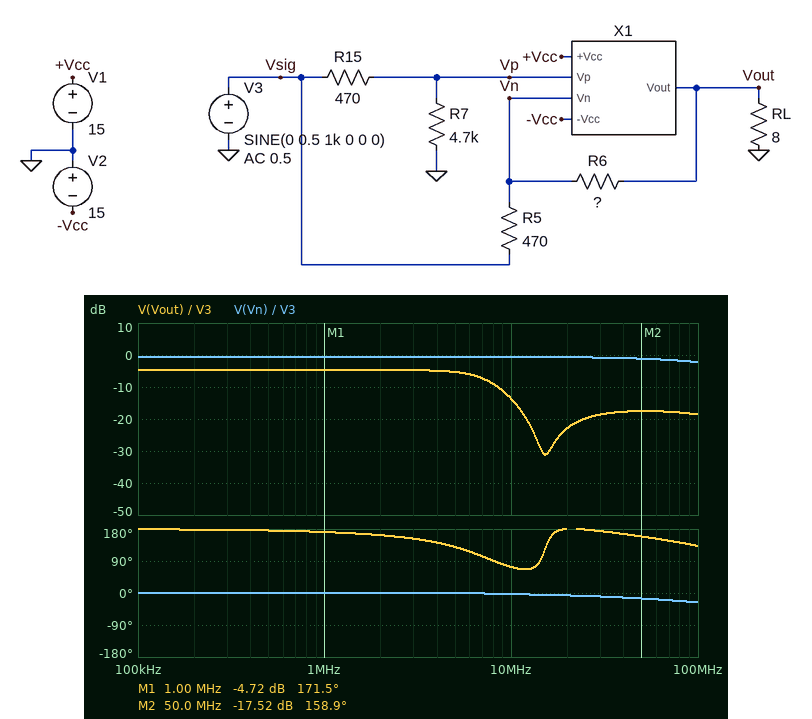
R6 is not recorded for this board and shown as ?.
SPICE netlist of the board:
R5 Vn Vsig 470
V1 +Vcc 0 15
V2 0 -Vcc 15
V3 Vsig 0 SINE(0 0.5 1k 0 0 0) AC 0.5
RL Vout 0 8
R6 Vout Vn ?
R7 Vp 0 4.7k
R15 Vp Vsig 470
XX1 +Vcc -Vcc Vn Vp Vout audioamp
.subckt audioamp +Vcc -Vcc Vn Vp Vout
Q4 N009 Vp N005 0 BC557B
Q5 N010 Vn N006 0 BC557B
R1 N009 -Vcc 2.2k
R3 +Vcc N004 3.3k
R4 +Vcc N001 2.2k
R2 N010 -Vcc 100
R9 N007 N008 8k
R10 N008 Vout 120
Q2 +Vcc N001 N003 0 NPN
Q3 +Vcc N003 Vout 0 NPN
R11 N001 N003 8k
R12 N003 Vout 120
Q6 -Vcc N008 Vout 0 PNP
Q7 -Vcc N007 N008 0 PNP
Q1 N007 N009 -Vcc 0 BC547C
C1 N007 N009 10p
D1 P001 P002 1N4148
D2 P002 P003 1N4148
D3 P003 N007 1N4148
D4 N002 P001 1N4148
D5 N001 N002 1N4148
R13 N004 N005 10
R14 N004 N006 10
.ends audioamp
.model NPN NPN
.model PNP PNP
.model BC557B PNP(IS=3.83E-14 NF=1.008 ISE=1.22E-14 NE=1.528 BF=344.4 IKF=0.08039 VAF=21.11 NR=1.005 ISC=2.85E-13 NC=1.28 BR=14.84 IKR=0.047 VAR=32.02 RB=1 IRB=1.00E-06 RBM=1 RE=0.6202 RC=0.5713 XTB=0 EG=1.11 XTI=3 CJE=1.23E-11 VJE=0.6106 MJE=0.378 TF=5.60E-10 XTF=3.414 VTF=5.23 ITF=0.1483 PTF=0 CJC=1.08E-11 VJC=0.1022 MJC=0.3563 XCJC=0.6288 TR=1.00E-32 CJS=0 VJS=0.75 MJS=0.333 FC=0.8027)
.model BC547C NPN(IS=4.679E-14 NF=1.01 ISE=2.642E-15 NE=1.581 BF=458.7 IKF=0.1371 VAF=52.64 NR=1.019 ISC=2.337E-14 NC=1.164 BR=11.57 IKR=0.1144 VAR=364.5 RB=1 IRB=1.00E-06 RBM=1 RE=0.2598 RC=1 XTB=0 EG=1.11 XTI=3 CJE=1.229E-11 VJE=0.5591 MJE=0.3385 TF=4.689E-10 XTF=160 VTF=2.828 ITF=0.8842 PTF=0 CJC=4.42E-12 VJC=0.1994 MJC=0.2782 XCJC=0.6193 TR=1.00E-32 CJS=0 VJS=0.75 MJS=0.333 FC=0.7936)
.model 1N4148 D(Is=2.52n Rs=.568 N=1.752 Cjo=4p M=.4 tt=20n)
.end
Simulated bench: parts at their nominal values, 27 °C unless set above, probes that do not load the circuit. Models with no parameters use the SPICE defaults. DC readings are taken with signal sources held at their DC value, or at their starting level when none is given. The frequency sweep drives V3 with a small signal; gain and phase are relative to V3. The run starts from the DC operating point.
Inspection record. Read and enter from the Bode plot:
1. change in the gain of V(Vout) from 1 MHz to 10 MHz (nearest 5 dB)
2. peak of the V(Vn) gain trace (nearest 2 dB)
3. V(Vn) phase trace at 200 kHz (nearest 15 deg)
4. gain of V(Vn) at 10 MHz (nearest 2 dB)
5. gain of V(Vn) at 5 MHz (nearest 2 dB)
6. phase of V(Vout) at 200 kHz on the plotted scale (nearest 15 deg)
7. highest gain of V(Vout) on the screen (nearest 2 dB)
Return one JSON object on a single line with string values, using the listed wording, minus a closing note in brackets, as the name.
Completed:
{"change in the gain of V(Vout) from 1 MHz to 10 MHz": "-10 dB", "peak of the V(Vn) gain trace": "0 dB", "V(Vn) phase trace at 200 kHz": "0 deg", "gain of V(Vn) at 10 MHz": "0 dB", "gain of V(Vn) at 5 MHz": "0 dB", "phase of V(Vout) at 200 kHz on the plotted scale": "180 deg", "highest gain of V(Vout) on the screen": "-4 dB"}
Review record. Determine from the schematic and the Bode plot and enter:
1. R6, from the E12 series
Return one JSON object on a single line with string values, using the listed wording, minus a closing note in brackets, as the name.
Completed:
{"R6, from the E12 series": "8.2 kΩ"}
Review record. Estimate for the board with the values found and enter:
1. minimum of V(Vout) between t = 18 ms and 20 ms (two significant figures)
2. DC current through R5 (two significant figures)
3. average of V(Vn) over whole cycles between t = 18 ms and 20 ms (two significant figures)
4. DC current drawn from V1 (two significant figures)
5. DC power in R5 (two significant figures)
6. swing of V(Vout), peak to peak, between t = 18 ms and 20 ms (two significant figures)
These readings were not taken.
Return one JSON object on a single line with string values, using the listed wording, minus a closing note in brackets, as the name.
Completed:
{"minimum of V(Vout) between t = 18 ms and 20 ms": "-2.3 V", "DC current through R5": "230 µA", "average of V(Vn) over whole cycles between t = 18 ms and 20 ms": "-110 mV", "DC current drawn from V1": "21 mA", "DC power in R5": "24 µW", "swing of V(Vout), peak to peak, between t = 18 ms and 20 ms": "580 mV"}
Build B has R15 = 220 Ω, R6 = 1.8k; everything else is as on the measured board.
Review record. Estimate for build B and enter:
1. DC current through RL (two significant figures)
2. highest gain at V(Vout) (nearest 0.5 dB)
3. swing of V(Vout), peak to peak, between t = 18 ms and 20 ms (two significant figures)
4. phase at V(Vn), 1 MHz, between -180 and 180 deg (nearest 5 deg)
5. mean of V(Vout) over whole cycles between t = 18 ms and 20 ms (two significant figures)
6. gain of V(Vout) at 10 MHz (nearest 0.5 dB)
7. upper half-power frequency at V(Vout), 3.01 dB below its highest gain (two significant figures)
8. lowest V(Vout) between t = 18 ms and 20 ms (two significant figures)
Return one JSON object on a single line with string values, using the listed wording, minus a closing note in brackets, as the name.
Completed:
{"DC current through RL": "66 mA", "highest gain at V(Vout)": "4.0 dB", "swing of V(Vout), peak to peak, between t = 18 ms and 20 ms": "810 mV", "phase at V(Vn), 1 MHz, between -180 and 180 deg": "0 deg", "mean of V(Vout) over whole cycles between t = 18 ms and 20 ms": "-530 mV", "gain of V(Vout) at 10 MHz": "0.5 dB", "upper half-power frequency at V(Vout), 3.01 dB below its highest gain": "24 MHz", "lowest V(Vout) between t = 18 ms and 20 ms": "-930 mV"}
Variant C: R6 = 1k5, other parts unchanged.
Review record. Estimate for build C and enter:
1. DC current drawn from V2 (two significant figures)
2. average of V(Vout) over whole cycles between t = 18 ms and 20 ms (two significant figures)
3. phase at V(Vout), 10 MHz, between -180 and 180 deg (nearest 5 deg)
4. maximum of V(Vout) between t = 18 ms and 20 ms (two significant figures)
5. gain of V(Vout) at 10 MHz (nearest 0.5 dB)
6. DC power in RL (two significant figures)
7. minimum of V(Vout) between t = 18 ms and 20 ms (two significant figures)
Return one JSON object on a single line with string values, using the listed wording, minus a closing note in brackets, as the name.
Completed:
{"DC current drawn from V2": "80 mA", "average of V(Vout) over whole cycles between t = 18 ms and 20 ms": "-460 mV", "phase at V(Vout), 10 MHz, between -180 and 180 deg": "-35 deg", "maximum of V(Vout) between t = 18 ms and 20 ms": "-140 mV", "gain of V(Vout) at 10 MHz": "0 dB", "DC power in RL": "26 mW", "minimum of V(Vout) between t = 18 ms and 20 ms": "-780 mV"}
